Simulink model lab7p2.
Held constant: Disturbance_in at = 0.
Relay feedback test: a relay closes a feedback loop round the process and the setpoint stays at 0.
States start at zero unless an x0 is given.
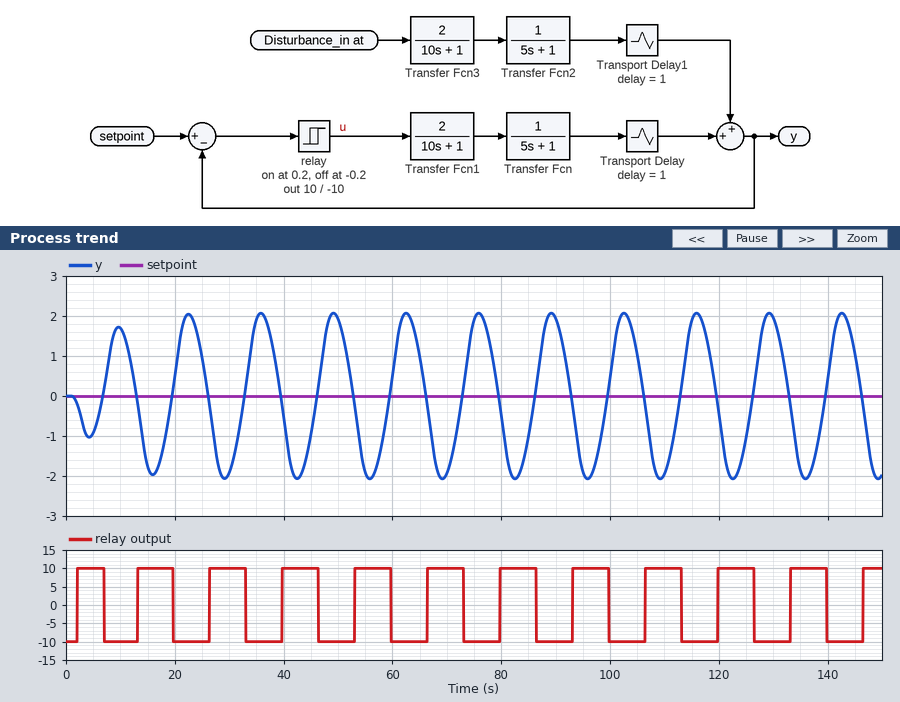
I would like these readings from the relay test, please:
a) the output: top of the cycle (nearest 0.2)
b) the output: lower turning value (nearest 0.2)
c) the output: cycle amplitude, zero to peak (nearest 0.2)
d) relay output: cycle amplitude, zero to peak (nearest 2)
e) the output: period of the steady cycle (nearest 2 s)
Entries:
2.0
-2.0
2.0
10
14 s
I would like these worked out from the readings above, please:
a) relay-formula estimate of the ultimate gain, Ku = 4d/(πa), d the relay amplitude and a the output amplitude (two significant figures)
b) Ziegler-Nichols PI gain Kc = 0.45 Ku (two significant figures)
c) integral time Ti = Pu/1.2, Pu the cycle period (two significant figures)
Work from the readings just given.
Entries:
6.4
2.9
12 s
